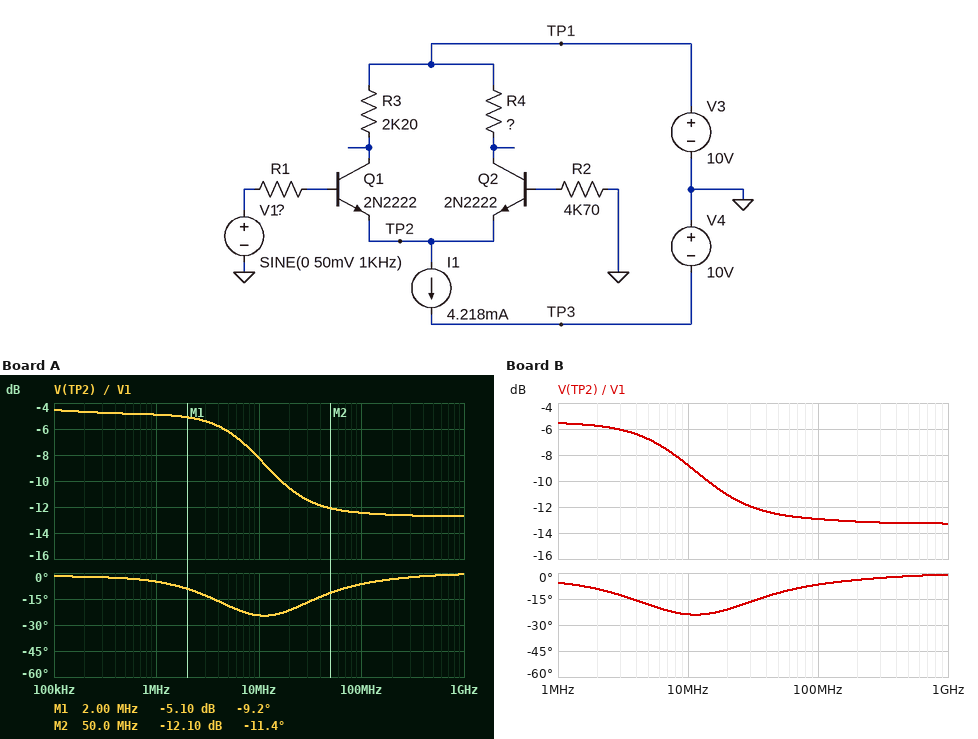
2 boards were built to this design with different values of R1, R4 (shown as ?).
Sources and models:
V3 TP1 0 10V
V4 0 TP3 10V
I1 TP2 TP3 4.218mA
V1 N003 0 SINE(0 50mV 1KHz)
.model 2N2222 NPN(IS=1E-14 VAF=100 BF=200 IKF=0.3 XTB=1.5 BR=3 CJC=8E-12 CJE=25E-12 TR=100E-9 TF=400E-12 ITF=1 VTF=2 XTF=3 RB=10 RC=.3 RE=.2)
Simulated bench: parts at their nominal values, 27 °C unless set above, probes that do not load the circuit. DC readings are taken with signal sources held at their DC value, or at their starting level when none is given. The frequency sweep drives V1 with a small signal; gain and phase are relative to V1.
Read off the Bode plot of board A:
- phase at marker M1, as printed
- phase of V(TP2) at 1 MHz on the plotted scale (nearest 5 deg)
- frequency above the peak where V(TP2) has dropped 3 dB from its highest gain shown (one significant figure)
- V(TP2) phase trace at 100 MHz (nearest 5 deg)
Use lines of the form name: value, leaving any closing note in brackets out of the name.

phase at marker M1, as printed: -9.2 deg
phase of V(TP2) at 1 MHz on the plotted scale: -5 deg
frequency above the peak where V(TP2) has dropped 3 dB from its highest gain shown: 8 MHz
V(TP2) phase trace at 100 MHz: -5 deg
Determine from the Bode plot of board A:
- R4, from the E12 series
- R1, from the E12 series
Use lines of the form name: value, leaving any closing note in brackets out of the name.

R4, from the E12 series: 1.8 kΩ
R1, from the E12 series: 2.7 kΩ
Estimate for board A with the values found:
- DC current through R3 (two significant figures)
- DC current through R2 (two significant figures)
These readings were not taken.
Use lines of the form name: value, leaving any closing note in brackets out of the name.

DC current through R3: 2.4 mA
DC current through R2: 8.4 µA
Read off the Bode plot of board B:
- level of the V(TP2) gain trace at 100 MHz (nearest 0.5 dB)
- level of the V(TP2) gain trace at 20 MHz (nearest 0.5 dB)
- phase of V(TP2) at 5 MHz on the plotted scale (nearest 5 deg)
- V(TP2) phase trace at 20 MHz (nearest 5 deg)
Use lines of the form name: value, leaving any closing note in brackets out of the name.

level of the V(TP2) gain trace at 100 MHz: -13.0 dB
level of the V(TP2) gain trace at 20 MHz: -11.0 dB
phase of V(TP2) at 5 MHz on the plotted scale: -20 deg
V(TP2) phase trace at 20 MHz: -20 deg
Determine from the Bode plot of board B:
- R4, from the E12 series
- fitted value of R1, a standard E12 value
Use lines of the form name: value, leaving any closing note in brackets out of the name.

R4, from the E12 series: 1.5 kΩ
fitted value of R1, a standard E12 value: 2.7 kΩ
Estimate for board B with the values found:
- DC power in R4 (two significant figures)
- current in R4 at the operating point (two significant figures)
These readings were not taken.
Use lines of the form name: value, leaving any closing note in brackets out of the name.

DC power in R4: 4.8 mW
current in R4 at the operating point: 1.8 mA
